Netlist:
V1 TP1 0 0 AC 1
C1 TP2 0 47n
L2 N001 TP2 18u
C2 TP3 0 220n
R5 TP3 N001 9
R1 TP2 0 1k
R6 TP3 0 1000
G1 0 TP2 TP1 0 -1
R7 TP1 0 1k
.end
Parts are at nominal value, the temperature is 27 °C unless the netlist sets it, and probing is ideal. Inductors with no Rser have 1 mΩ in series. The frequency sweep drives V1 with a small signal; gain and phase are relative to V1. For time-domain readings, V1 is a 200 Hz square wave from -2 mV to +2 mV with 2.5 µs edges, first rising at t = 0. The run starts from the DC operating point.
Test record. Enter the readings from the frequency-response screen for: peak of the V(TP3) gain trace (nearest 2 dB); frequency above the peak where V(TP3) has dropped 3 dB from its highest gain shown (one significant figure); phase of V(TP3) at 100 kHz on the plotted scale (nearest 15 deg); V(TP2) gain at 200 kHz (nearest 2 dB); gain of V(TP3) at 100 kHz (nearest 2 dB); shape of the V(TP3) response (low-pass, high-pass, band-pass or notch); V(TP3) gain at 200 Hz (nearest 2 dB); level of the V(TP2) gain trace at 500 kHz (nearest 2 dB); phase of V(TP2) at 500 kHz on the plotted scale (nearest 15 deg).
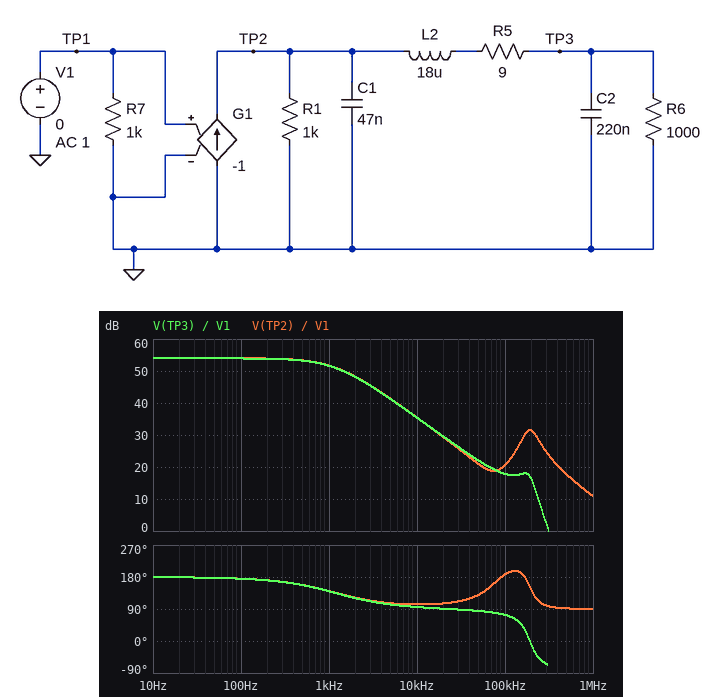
54 dB
1 kHz
75 deg
32 dB
18 dB
low-pass
54 dB
18 dB
90 deg
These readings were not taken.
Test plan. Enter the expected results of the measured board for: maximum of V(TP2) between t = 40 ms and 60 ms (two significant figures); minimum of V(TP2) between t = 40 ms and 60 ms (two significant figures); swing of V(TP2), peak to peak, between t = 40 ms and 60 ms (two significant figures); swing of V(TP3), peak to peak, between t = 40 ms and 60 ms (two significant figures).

1.0 V
-1.0 V
2.0 V
2.0 V
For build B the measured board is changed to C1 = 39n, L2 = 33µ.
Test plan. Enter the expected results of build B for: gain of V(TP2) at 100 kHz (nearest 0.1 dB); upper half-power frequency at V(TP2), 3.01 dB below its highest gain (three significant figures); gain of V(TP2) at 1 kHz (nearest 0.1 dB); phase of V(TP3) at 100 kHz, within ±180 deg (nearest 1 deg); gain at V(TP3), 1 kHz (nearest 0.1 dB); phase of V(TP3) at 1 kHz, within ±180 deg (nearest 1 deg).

27.1 dB
1.23 kHz
51.8 dB
71 deg
51.7 dB
141 deg
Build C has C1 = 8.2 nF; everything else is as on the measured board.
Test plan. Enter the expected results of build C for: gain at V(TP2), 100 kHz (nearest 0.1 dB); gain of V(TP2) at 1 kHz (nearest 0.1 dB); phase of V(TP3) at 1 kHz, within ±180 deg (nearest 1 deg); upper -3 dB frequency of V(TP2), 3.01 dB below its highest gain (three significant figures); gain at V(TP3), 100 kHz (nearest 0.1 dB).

20.0 dB
52.2 dB
144 deg
1.39 kHz
17.3 dB
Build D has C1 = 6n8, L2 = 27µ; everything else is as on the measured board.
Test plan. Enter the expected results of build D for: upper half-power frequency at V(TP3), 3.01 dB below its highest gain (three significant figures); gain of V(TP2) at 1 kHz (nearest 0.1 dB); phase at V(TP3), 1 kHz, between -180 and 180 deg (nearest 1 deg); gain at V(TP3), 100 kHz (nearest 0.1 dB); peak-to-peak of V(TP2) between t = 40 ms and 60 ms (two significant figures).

1.40 kHz
52.2 dB
144 deg
17.5 dB
2.0 V
